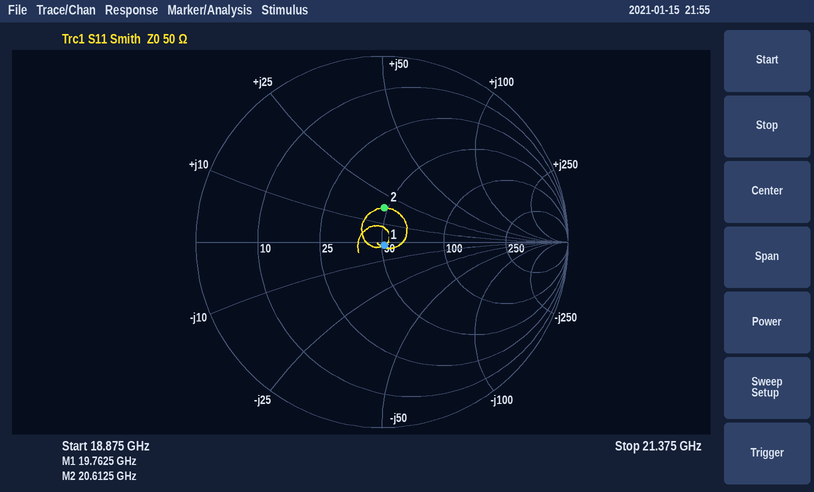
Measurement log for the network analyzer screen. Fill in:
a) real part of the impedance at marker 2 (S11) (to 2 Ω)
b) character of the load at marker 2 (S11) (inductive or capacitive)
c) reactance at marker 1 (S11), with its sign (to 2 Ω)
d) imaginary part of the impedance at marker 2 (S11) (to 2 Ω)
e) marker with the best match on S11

48 Ω
inductive
-2 Ω
+18 Ω
marker 1
